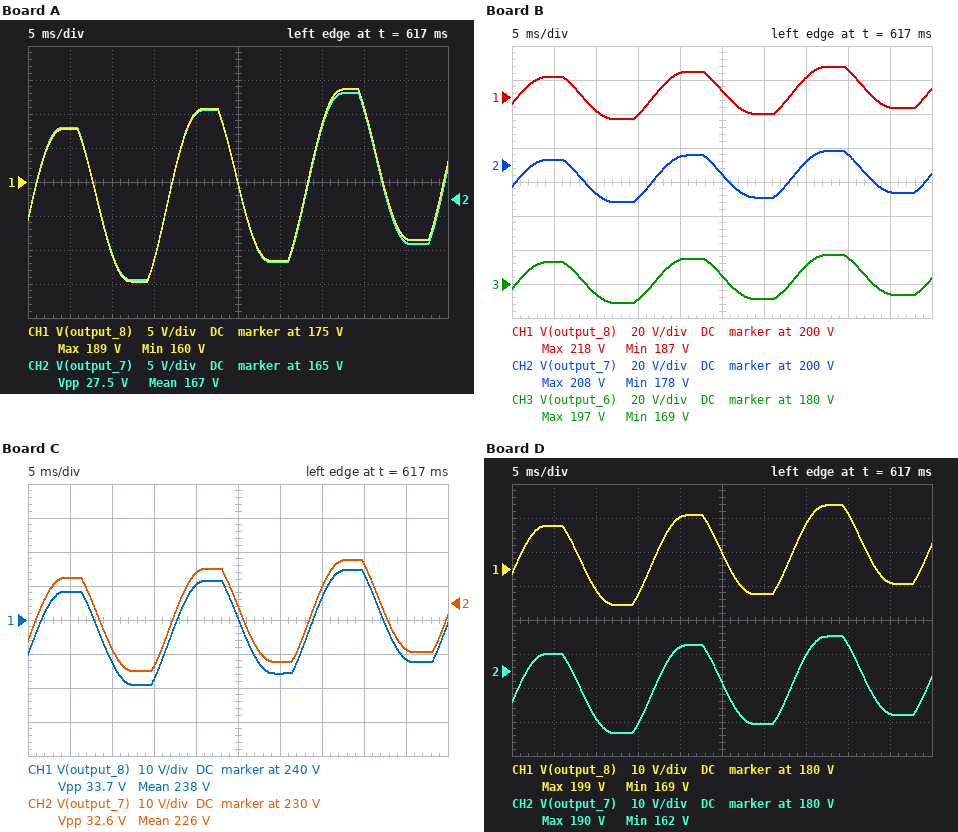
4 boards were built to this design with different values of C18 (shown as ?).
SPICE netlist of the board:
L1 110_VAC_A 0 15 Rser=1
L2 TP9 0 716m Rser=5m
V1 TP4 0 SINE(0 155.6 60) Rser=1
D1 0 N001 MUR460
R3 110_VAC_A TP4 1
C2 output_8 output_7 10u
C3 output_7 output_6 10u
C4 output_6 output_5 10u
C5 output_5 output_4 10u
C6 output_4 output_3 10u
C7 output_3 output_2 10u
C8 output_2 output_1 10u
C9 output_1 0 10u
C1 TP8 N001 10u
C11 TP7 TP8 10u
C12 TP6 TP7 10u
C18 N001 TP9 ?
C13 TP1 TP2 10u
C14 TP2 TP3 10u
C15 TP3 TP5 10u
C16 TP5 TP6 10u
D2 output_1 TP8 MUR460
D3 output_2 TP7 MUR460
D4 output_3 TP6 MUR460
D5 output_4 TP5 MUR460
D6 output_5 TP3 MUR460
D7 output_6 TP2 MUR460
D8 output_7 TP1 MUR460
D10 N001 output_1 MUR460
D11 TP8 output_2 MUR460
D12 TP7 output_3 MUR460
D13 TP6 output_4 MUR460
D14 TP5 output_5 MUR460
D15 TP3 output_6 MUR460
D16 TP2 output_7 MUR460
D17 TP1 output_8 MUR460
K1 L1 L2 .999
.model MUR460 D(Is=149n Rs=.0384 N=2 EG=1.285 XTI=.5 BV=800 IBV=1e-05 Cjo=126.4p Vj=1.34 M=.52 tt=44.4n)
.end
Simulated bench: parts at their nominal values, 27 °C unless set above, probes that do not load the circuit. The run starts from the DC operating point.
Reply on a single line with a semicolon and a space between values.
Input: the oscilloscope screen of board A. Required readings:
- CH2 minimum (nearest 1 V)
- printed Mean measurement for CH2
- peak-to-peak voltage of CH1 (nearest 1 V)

153 V; 167 V; 28 V
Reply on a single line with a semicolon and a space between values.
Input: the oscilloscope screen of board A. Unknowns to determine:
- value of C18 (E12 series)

3.3 µF
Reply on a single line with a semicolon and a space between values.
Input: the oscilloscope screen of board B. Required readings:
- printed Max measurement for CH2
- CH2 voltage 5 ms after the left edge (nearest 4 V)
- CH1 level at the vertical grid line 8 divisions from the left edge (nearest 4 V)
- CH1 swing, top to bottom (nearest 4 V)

208 V; 204 V; 216 V; 32 V
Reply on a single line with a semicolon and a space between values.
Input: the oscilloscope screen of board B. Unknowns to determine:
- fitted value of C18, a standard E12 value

5.6 µF
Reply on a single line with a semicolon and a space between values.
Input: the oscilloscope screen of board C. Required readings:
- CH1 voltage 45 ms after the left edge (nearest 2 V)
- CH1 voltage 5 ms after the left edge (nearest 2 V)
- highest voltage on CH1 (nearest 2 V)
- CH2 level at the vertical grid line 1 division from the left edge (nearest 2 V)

228 V; 248 V; 254 V; 238 V
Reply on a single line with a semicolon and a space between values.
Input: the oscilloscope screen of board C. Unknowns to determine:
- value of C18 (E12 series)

18 µF
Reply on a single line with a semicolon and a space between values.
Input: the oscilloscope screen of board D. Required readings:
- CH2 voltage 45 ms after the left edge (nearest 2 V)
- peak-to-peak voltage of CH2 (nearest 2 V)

168 V; 28 V
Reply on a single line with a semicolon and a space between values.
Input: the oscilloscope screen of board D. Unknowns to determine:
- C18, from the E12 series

3.9 µF
